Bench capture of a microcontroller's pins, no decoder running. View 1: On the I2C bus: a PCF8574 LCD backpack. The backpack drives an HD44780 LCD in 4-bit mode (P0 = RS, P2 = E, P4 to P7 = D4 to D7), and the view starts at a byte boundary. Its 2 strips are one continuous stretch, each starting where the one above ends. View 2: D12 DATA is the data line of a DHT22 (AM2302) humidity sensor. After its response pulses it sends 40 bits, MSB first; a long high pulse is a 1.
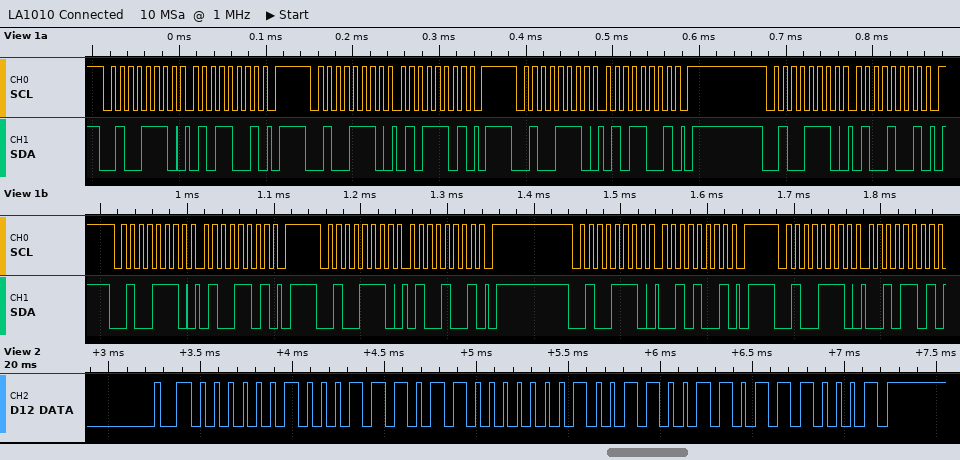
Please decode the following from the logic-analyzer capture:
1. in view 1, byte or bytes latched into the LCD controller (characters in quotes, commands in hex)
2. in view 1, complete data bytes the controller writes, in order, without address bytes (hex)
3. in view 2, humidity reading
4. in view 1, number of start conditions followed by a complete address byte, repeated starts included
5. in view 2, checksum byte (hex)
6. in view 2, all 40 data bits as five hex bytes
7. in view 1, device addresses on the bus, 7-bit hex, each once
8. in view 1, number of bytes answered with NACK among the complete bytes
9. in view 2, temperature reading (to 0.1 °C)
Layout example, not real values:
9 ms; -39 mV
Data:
'T'; 59 5D 59 49 4D 49 29 2D; 57.1 %; 8; 0x71; 02 3B 01 33 71; 0x27; 0; 30.7 °C
